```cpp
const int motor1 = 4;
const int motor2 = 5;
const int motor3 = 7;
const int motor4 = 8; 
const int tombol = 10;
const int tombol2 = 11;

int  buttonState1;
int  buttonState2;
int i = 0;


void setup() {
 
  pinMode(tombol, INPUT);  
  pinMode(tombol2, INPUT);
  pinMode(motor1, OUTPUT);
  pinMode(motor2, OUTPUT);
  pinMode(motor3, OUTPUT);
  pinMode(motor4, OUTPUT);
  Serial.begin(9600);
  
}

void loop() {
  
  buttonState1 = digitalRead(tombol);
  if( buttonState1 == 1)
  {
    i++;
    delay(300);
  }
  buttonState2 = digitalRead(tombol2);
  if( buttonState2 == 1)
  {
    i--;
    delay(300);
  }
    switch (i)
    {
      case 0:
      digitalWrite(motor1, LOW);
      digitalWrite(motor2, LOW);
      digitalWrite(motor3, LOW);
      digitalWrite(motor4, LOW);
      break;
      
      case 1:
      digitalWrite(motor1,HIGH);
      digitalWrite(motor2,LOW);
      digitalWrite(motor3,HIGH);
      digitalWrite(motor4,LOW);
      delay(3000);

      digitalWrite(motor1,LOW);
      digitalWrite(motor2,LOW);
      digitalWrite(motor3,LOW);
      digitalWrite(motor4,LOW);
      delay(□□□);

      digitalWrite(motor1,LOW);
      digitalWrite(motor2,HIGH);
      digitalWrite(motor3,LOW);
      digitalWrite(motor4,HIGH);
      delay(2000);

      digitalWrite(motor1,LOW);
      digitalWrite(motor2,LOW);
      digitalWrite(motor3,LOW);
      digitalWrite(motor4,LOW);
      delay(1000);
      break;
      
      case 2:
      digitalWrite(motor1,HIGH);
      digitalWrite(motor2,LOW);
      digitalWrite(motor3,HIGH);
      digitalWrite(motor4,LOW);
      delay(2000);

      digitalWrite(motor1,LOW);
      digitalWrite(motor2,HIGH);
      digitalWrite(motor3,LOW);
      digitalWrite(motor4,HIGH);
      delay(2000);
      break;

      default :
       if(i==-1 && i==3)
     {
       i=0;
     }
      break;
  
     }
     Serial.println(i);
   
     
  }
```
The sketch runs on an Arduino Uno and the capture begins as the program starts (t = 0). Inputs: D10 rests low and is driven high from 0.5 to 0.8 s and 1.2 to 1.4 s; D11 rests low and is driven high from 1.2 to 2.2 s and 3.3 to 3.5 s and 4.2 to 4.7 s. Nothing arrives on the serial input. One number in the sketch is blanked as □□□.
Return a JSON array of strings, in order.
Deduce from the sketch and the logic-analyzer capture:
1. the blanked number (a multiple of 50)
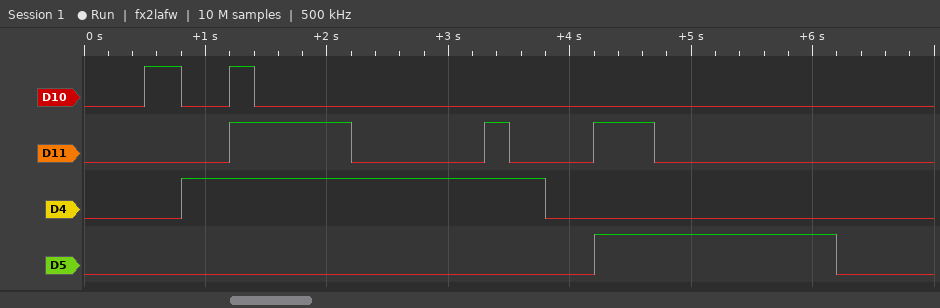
["400"]
